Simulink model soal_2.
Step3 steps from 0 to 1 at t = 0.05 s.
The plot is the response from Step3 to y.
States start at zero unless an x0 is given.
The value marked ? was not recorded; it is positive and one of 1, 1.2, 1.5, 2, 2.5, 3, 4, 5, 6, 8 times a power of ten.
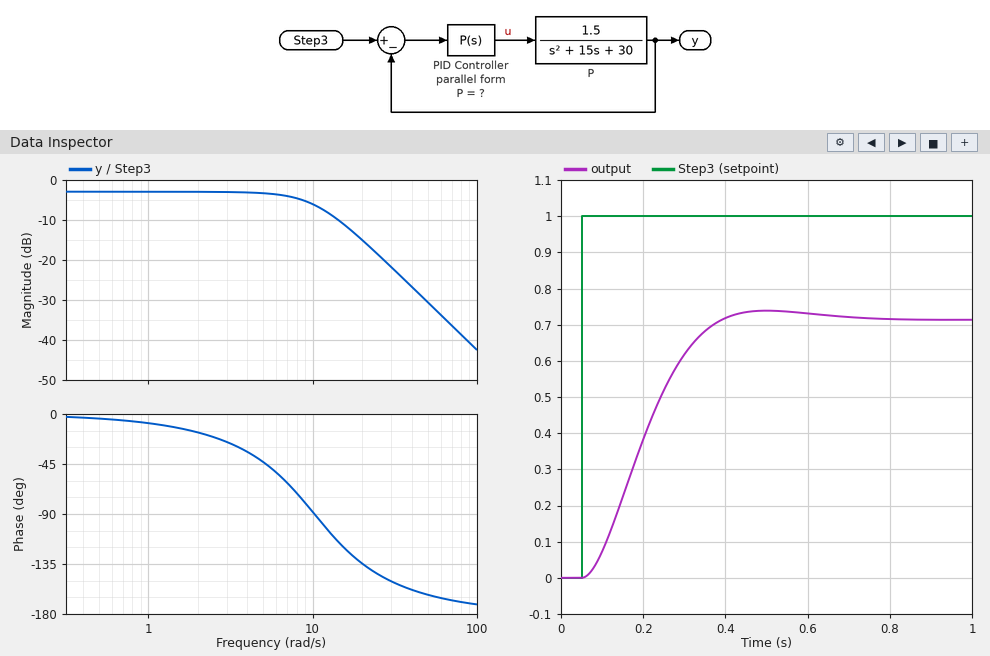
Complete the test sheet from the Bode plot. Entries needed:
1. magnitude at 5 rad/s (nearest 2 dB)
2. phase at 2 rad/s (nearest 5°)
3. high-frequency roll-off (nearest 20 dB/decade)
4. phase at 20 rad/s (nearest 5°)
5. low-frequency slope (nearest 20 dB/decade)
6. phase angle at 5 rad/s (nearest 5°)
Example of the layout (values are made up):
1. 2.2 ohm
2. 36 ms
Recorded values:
1. -4 dB
2. -15°
3. -40 dB/decade
4. -135°
5. 0 dB/decade
6. -45°
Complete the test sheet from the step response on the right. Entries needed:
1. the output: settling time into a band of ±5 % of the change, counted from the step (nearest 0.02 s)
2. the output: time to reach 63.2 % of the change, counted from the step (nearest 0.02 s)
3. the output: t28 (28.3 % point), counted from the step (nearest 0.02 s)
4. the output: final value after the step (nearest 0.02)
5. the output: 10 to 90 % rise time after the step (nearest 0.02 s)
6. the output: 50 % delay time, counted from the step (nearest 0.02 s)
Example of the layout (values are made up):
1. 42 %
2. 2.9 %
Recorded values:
1. 0.30 s
2. 0.18 s
3. 0.10 s
4. 0.72
5. 0.22 s
6. 0.14 s
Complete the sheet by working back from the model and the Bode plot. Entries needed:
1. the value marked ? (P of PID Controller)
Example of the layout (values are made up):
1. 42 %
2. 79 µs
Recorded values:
1. 50
